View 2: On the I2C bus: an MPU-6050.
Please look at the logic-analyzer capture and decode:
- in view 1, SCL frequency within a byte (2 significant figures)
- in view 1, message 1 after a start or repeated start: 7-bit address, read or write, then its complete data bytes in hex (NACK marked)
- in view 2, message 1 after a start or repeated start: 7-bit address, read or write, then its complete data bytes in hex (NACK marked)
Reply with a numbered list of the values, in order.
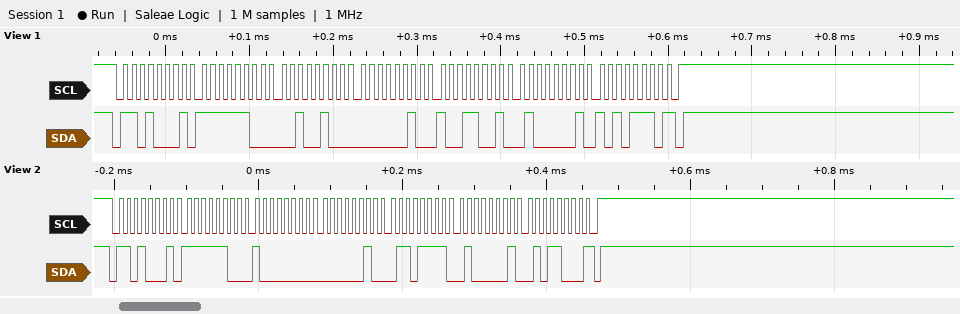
1. 100 kHz
2. 0x68 read: FC 24 02 99 41 AE NACK
3. 0x68 read: FC 80 02 6F 41 58 NACK
